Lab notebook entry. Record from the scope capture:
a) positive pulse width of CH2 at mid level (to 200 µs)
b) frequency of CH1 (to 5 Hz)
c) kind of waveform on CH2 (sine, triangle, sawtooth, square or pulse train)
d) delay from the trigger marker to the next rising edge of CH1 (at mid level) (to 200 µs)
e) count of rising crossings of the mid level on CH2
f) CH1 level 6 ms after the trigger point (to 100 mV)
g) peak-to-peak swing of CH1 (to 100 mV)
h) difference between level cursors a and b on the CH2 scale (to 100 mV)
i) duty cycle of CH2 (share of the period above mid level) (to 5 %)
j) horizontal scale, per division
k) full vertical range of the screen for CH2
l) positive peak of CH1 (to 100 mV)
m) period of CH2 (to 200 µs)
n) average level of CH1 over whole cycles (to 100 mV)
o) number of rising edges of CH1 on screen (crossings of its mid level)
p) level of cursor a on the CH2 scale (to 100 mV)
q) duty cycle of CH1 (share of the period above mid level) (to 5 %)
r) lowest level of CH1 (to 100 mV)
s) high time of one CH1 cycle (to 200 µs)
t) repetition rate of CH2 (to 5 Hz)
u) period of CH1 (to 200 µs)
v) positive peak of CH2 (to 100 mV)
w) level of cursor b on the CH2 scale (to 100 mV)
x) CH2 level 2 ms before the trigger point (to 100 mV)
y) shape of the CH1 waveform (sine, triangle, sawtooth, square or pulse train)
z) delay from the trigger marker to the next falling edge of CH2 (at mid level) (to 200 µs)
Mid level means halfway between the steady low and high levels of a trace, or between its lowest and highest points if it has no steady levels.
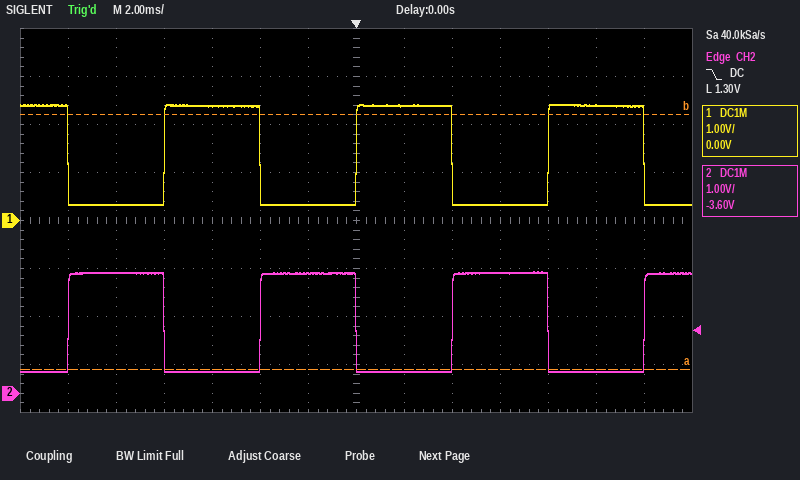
4.0 ms
125 Hz
square
8.0 ms
4
300 mV
2.1 V
5.3 V
50 %
2 ms
8 V
2.4 V
8.0 ms
1.4 V
3
500 mV
50 %
300 mV
4.0 ms
125 Hz
8.0 ms
2.5 V
5.8 V
2.5 V
square
8.0 ms
